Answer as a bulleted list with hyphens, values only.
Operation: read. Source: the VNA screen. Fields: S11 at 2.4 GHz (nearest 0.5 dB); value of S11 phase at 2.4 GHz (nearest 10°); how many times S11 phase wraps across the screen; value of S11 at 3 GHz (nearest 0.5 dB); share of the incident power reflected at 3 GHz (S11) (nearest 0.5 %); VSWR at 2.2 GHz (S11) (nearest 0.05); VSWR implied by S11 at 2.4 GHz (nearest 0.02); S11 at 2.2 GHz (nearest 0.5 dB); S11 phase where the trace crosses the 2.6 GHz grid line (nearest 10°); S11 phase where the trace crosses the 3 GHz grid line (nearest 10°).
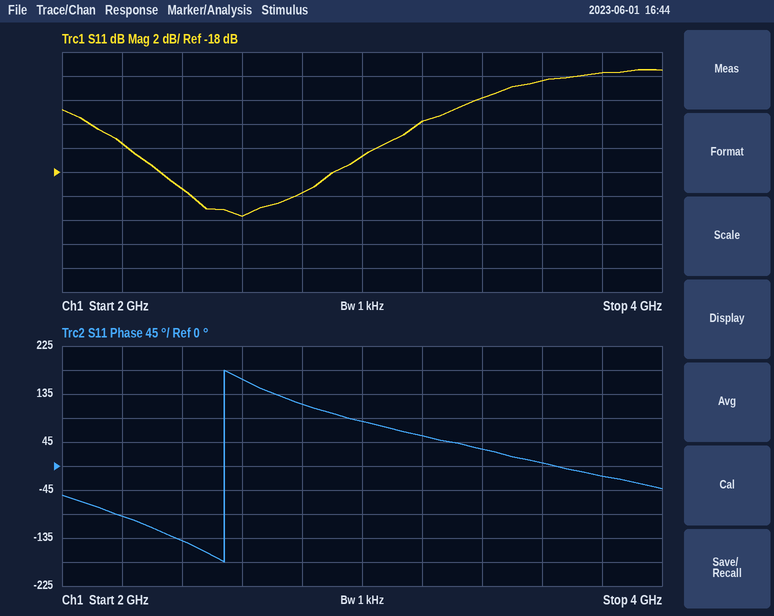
- -19.5 dB
- -140°
- 1
- -16.5 dB
- 2.0 %
- 1.40
- 1.24
- -15.5 dB
- 160°
- 80°
